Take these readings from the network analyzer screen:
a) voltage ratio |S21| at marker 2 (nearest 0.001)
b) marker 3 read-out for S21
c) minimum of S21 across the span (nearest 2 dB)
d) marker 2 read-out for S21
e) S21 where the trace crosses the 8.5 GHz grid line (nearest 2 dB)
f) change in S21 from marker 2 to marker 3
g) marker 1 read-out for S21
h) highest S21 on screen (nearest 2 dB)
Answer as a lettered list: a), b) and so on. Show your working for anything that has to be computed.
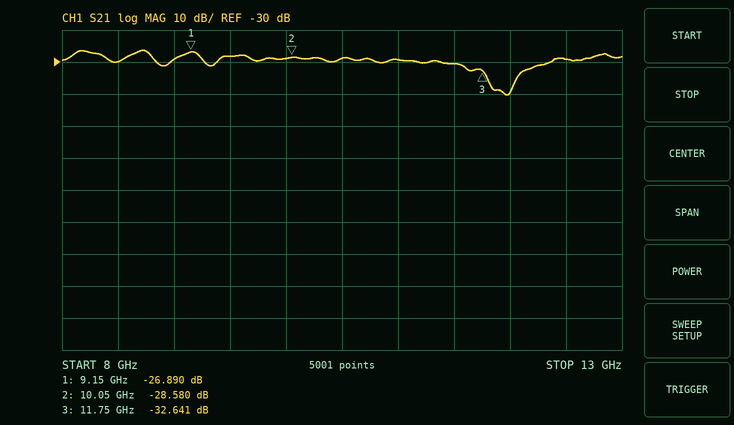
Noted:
a) 10^(-28.58/20) ≈ 0.037
b) -32.641 dB
c) -40 dB
d) -28.580 dB
e) -30 dB
f) -32.641 − (-28.58) = -4.061 dB
g) -26.890 dB
h) -26 dB
